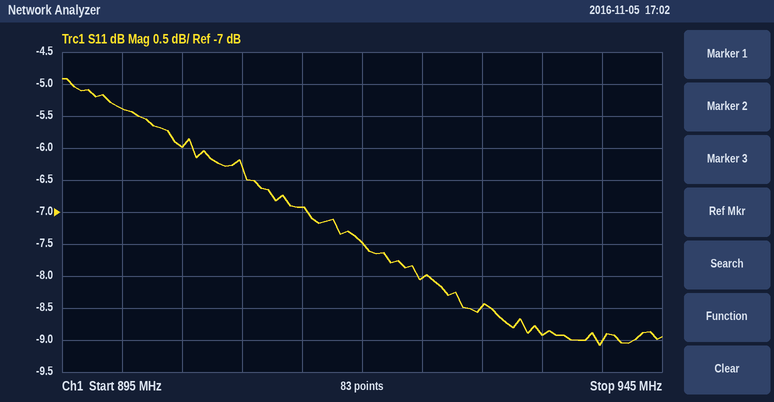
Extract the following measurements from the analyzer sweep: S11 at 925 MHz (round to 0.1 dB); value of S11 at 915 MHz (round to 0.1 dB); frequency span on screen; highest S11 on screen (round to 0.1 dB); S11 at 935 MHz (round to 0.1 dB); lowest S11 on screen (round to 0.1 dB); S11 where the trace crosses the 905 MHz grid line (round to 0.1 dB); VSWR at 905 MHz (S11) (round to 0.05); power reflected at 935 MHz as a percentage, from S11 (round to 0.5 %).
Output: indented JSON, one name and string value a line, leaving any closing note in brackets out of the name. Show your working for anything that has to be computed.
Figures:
{
  "S11 at 925 MHz": "-8.0 dB",
  "value of S11 at 915 MHz": "-6.9 dB",
  "frequency span on screen": "50 MHz",
  "highest S11 on screen": "-4.9 dB",
  "S11 at 935 MHz": "-8.9 dB",
  "lowest S11 on screen": "-9.1 dB",
  "S11 where the trace crosses the 905 MHz grid line": "-6.0 dB",
  "VSWR at 905 MHz (S11)": "|Γ| = 10^(-6/20) = 0.5012; VSWR = (1 + 0.5012)/(1 − 0.5012) ≈ 3.01, so 3.00 to the nearest 0.05",
  "power reflected at 935 MHz as a percentage, from S11": "10^(-8.9/10) ≈ 12.9 %, so 13.0 % to the nearest 0.5 %"
}
